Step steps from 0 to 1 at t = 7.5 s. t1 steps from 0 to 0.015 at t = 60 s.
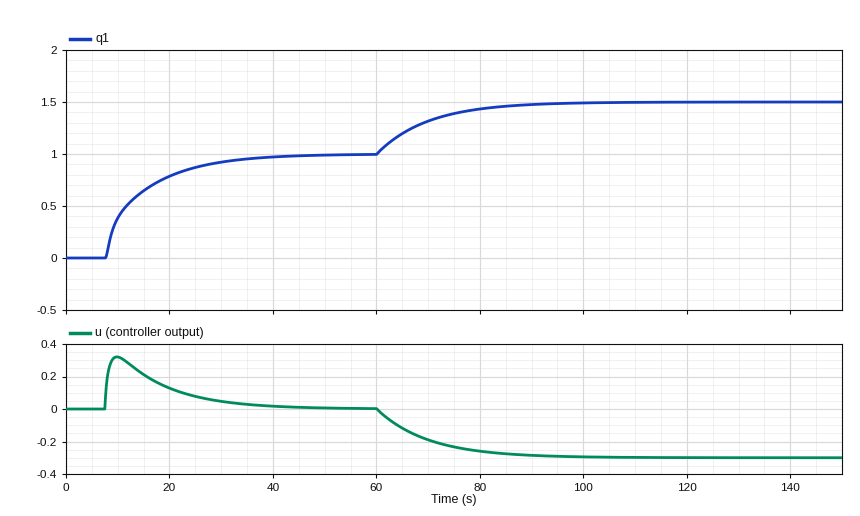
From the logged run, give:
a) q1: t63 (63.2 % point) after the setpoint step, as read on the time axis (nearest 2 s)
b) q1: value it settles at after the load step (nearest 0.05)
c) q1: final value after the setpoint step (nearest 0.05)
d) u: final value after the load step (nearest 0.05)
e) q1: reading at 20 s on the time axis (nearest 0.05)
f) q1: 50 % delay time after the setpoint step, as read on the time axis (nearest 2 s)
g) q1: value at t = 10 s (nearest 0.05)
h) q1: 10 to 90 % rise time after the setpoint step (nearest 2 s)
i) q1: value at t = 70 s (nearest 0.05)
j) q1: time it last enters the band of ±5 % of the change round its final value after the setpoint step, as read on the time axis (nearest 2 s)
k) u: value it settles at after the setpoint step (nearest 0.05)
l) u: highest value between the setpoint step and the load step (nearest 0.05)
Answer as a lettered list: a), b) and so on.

a) 14 s
b) 1.50
c) 1.00
d) -0.30
e) 0.80
f) 12 s
g) 0.40
h) 20 s
i) 1.30
j) 34 s
k) 0.00
l) 0.30
